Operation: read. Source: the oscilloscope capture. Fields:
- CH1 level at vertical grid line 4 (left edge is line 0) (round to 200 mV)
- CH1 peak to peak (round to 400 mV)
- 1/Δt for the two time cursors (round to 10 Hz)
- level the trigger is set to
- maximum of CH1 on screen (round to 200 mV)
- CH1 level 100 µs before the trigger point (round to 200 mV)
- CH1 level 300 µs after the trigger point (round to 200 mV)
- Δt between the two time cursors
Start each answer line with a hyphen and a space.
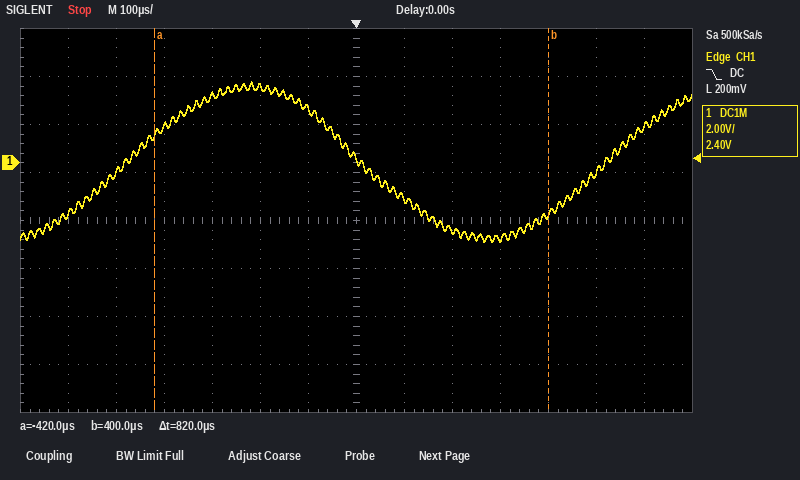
- 2.8 V
- 6.8 V
- 1.22 kHz
- 200 mV
- 3.4 V
- 2.2 V
- -3.2 V
- 820 µs
